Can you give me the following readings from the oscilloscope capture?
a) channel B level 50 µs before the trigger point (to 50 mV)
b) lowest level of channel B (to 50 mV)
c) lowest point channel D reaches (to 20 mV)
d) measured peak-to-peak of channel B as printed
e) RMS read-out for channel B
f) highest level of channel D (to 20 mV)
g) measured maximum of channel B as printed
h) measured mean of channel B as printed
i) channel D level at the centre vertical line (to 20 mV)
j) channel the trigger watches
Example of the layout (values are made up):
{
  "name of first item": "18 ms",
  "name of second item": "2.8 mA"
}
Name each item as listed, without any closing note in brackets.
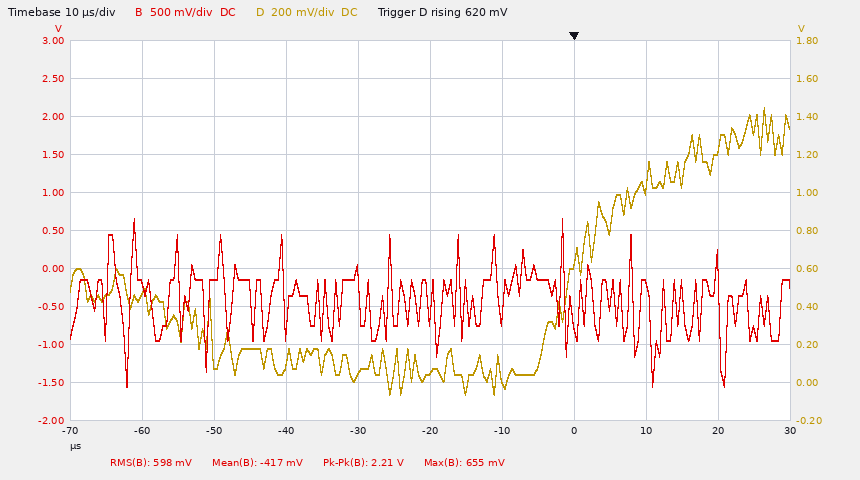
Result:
{
  "channel B level 50 µs before the trigger point": "-150 mV",
  "lowest level of channel B": "-1.55 V",
  "lowest point channel D reaches": "-60 mV",
  "measured peak-to-peak of channel B as printed": "2.21 V",
  "RMS read-out for channel B": "598 mV",
  "highest level of channel D": "1.44 V",
  "measured maximum of channel B as printed": "655 mV",
  "measured mean of channel B as printed": "-417 mV",
  "channel D level at the centre vertical line": "60 mV",
  "channel the trigger watches": "channel D"
}
